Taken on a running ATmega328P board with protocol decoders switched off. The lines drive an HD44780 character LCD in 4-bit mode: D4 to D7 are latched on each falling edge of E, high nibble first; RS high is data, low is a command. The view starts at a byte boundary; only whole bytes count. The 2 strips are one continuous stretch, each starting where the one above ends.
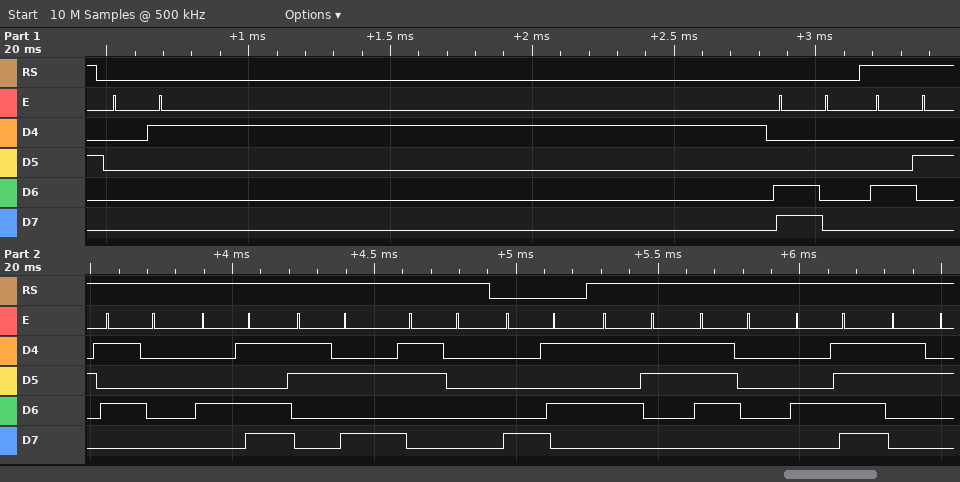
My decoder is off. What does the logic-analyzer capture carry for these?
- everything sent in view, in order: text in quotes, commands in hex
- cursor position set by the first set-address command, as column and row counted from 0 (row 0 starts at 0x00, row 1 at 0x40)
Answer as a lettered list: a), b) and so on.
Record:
a) 0x01 0xC0 "BPM:0" 0x85 "SpO2"
b) column 0, row 1
